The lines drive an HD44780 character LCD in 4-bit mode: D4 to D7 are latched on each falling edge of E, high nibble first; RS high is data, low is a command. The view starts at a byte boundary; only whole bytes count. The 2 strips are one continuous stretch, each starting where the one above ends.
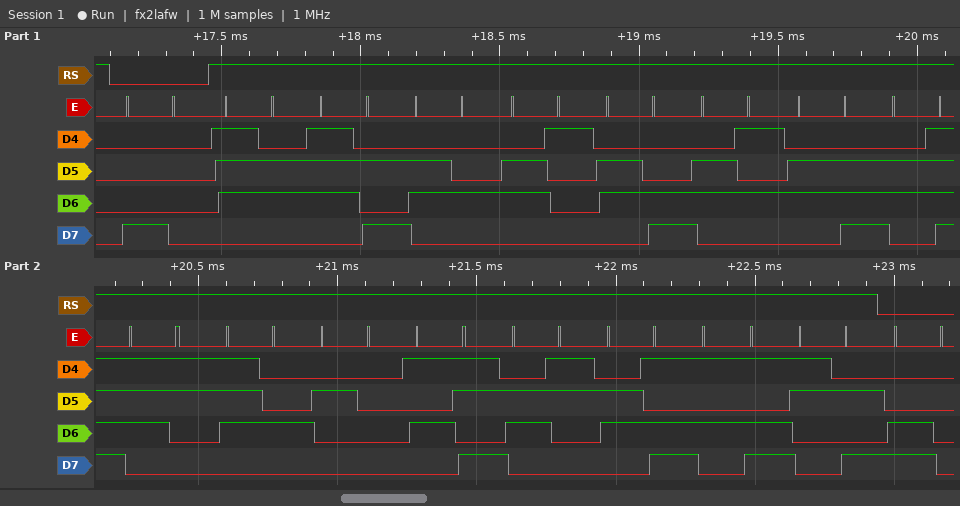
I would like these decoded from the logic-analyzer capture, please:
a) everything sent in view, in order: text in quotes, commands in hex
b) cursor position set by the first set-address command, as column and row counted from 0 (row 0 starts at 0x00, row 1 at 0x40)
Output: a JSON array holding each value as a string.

["0x80 \"vzdalenost [cm]:\" 0xC0", "column 0, row 0"]
